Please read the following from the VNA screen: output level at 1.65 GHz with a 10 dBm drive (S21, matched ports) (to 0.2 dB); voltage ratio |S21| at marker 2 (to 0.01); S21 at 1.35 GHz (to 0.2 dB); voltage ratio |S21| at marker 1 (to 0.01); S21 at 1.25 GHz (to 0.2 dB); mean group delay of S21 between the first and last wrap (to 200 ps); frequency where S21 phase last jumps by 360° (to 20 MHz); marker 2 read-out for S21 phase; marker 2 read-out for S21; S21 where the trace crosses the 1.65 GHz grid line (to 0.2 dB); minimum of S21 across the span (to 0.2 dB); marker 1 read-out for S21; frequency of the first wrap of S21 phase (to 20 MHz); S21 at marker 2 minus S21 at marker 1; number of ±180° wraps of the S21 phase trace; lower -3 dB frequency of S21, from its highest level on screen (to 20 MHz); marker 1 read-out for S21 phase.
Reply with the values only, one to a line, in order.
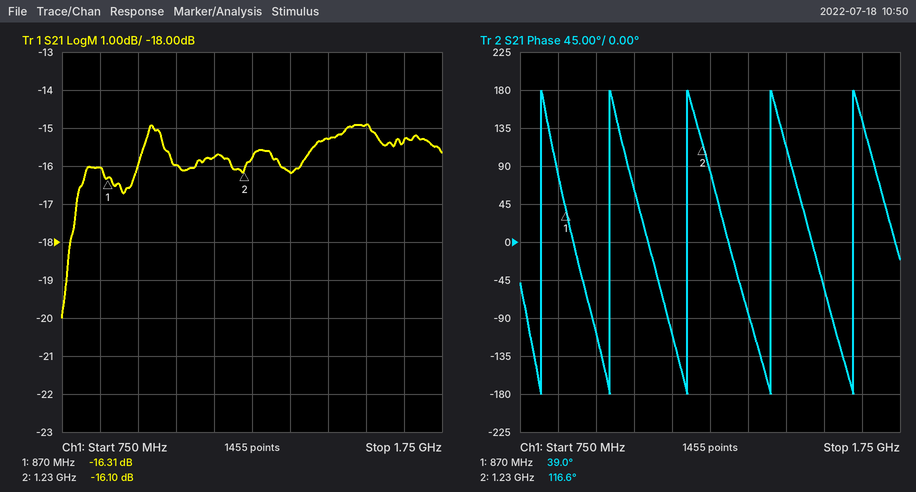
-5.4 dBm
0.16
-16.2 dB
0.15
-15.8 dB
4.8 ns
1.62 GHz
116.6°
-16.10 dB
-15.4 dB
-20.0 dB
-16.31 dB
800 MHz
0.21 dB
5
780 MHz
39.0°
